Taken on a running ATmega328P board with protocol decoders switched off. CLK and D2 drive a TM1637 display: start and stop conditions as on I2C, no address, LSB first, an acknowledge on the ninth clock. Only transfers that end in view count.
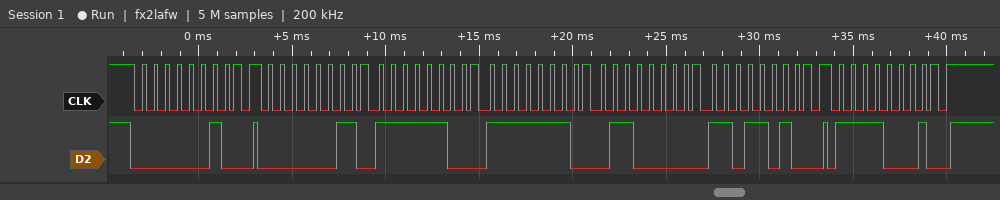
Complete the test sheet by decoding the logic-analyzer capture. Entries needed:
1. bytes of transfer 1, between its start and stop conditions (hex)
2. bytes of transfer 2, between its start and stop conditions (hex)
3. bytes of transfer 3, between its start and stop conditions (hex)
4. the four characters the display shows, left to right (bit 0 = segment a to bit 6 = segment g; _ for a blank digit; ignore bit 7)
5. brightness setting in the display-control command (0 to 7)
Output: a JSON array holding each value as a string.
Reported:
["40", "C0 3F 7F 06 5B", "8F", "0812", "7"]
